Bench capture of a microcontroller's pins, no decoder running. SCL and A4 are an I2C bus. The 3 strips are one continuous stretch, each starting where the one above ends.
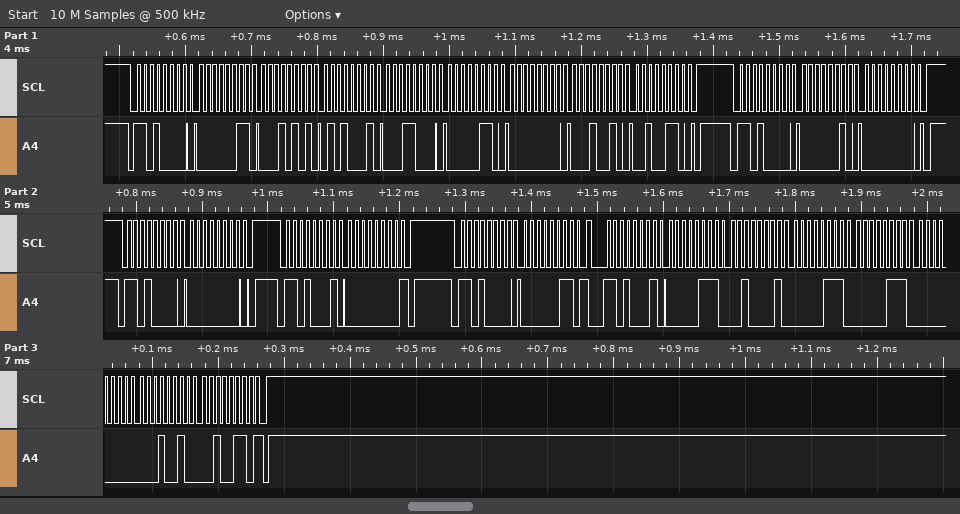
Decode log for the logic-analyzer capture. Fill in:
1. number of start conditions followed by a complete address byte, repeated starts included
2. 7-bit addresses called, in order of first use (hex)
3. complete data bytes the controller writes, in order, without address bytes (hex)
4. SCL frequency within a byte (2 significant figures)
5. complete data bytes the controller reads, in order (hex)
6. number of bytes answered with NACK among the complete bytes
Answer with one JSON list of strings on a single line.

["6", "0x68", "03 15 51 18 06 00 12 26 02 00 00 03", "100 kHz", "00 07 21 07 07 00 12 26", "2"]
